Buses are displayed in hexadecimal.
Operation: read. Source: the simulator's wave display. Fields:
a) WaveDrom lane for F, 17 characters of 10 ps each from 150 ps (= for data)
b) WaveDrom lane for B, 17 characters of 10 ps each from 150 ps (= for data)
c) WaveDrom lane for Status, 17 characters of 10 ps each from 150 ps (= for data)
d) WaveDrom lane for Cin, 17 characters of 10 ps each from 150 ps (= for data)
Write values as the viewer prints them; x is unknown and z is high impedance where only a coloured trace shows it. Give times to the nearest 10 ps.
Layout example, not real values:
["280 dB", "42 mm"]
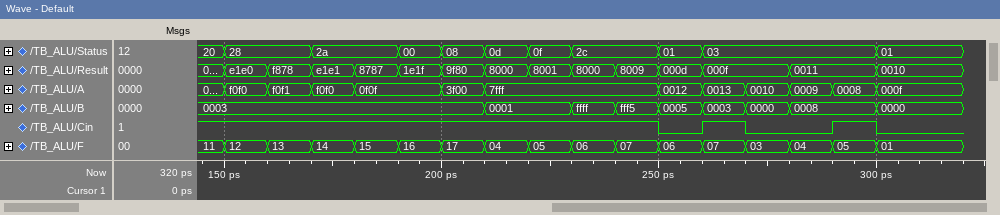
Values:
["{name: 'F', wave: '================.', data: '12 13 14 15 16 17 04 05 06 07 06 07 03 04 05 01'}", "{name: 'B', wave: '=.....=.======.=.', data: '0003 0001 ffff fff5 0005 0003 0000 0008 0000'}", "{name: 'Status', wave: '=.=.=====.==...=.', data: '28 2a 00 08 0d 0f 2c 01 03 01'}", "{name: 'Cin', wave: '1.........010.10.'}"]
